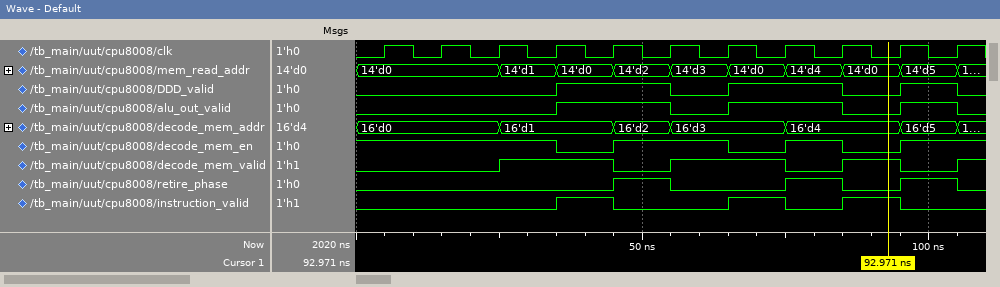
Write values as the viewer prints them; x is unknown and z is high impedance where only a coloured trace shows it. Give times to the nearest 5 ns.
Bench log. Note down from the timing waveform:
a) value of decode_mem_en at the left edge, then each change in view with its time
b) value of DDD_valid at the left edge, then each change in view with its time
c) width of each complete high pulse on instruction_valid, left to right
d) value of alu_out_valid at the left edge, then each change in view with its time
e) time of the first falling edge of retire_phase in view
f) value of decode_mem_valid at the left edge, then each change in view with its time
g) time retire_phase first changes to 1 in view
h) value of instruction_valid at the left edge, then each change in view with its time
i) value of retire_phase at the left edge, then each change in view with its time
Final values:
1, 0 at 35 ns, 1 at 45 ns, 0 at 65 ns, 1 at 75 ns, 0 at 85 ns, 1 at 95 ns
0, 1 at 35 ns, 0 at 55 ns, 1 at 65 ns, 0 at 85 ns, 1 at 95 ns, 0 at 105 ns
10 ns, 10 ns, 10 ns
0, 1 at 35 ns, 0 at 55 ns, 1 at 65 ns, 0 at 85 ns, 1 at 95 ns, 0 at 105 ns
55 ns
0, 1 at 25 ns, 0 at 45 ns, 1 at 55 ns, 0 at 75 ns, 1 at 85 ns, 0 at 95 ns, 1 at 105 ns
45 ns
0, 1 at 35 ns, 0 at 45 ns, 1 at 65 ns, 0 at 75 ns, 1 at 85 ns, 0 at 95 ns
0, 1 at 45 ns, 0 at 55 ns, 1 at 75 ns, 0 at 85 ns, 1 at 95 ns, 0 at 105 ns
